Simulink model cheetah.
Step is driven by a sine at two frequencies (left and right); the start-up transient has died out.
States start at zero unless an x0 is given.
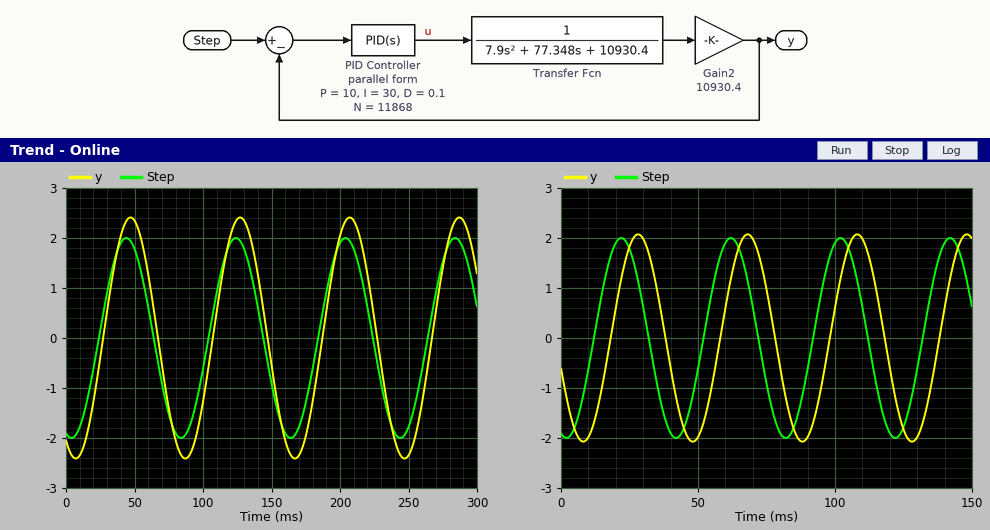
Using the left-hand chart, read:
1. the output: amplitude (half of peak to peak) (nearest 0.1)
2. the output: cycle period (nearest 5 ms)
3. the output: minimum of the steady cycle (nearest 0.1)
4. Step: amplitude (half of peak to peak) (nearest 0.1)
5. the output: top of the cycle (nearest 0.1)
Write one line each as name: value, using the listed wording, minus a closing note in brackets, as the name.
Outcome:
the output: amplitude (half of peak to peak): 2.4
the output: cycle period: 80 ms
the output: minimum of the steady cycle: -2.4
Step: amplitude (half of peak to peak): 2.0
the output: top of the cycle: 2.4
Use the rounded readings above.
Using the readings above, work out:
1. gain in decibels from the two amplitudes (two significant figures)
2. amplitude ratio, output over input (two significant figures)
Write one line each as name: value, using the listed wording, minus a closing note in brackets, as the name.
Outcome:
gain in decibels from the two amplitudes: 1.6 dB
amplitude ratio, output over input: 1.2
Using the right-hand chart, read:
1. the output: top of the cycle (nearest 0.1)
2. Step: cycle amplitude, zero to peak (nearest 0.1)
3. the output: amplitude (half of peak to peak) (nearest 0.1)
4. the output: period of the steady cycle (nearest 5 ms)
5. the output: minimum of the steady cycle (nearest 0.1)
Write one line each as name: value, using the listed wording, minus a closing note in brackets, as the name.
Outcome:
the output: top of the cycle: 2.1
Step: cycle amplitude, zero to peak: 2.0
the output: amplitude (half of peak to peak): 2.1
the output: period of the steady cycle: 40 ms
the output: minimum of the steady cycle: -2.1
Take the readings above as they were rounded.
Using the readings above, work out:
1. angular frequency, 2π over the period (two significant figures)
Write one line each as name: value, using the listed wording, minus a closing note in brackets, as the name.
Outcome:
angular frequency, 2π over the period: 0.16 rad/ms
